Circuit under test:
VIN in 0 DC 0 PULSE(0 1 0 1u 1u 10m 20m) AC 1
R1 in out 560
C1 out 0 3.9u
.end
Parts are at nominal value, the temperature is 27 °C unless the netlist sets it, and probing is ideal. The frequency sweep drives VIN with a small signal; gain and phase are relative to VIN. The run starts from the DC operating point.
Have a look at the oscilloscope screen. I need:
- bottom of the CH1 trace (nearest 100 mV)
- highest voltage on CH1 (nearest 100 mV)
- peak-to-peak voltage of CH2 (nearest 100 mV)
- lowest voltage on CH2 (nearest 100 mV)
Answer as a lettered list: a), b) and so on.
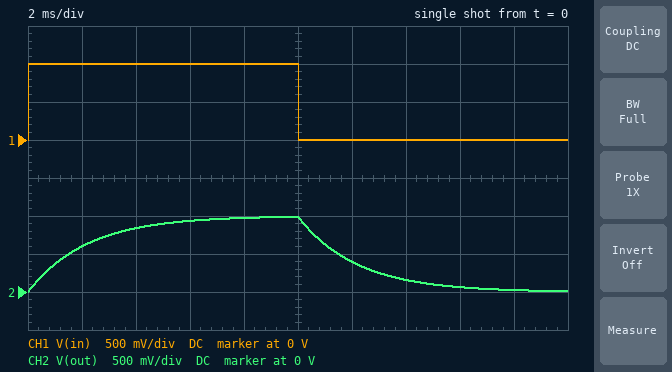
a) 0 V
b) 1.0 V
c) 1.0 V
d) 0 V
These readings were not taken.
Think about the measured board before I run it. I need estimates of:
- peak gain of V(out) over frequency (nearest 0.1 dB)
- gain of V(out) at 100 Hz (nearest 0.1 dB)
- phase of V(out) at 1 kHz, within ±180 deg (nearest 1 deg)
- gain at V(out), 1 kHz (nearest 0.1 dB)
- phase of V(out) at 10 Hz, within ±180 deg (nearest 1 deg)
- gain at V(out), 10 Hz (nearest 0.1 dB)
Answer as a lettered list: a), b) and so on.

a) 0 dB
b) -4.6 dB
c) -86 deg
d) -22.8 dB
e) -8 deg
f) -0.1 dB
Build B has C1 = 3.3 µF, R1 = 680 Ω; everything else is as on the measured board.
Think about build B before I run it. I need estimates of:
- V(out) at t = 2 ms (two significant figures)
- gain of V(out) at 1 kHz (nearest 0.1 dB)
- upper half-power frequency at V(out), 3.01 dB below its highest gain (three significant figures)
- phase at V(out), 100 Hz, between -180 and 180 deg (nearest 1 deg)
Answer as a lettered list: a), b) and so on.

a) 590 mV
b) -23.0 dB
c) 70.9 Hz
d) -55 deg
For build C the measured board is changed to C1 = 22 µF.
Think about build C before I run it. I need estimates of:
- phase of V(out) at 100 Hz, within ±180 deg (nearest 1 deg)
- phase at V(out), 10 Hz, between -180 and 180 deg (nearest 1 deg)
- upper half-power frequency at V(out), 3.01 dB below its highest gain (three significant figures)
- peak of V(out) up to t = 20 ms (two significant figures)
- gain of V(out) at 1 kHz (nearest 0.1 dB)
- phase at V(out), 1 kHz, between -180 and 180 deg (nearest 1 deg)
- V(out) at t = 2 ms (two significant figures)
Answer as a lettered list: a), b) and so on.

a) -83 deg
b) -38 deg
c) 12.9 Hz
d) 560 mV
e) -37.8 dB
f) -89 deg
g) 150 mV
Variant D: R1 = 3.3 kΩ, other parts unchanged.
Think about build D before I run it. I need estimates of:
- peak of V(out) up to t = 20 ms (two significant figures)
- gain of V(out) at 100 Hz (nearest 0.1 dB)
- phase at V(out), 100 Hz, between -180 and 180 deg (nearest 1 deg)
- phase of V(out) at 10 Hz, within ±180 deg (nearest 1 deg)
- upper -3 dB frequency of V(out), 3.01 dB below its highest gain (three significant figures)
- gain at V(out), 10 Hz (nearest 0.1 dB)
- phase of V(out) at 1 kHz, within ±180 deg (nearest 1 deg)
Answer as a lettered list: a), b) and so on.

a) 540 mV
b) -18.2 dB
c) -83 deg
d) -39 deg
e) 12.4 Hz
f) -2.2 dB
g) -89 deg
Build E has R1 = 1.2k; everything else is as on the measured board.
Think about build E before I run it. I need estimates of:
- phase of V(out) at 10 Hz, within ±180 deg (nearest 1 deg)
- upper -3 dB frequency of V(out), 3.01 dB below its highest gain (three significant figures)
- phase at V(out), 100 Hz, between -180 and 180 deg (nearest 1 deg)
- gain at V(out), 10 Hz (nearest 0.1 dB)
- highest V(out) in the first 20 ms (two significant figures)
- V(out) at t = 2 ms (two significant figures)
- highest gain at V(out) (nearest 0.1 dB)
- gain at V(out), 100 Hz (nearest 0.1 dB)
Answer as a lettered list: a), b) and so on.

a) -16 deg
b) 34.0 Hz
c) -71 deg
d) -0.4 dB
e) 880 mV
f) 350 mV
g) 0 dB
h) -9.8 dB
